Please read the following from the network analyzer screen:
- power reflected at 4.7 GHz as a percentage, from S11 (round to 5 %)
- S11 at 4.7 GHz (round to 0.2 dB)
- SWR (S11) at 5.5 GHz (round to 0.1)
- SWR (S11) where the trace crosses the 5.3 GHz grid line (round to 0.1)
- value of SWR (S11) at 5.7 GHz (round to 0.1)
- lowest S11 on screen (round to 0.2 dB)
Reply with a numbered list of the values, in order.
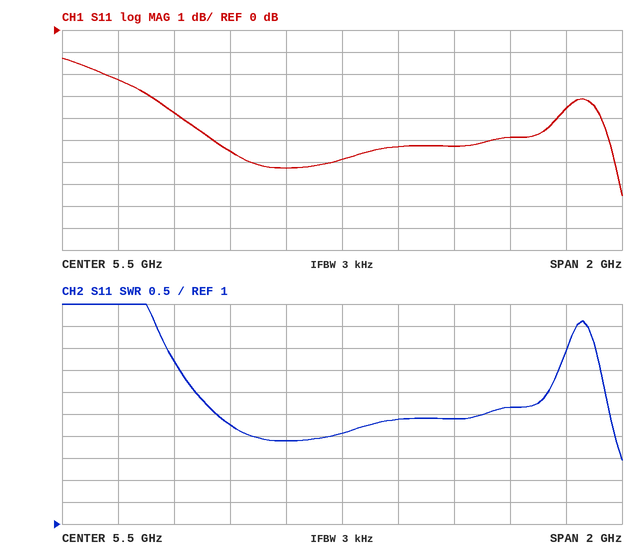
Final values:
1. 60 %
2. -2.2 dB
3. 3.1
4. 2.9
5. 3.4
6. -7.6 dB
